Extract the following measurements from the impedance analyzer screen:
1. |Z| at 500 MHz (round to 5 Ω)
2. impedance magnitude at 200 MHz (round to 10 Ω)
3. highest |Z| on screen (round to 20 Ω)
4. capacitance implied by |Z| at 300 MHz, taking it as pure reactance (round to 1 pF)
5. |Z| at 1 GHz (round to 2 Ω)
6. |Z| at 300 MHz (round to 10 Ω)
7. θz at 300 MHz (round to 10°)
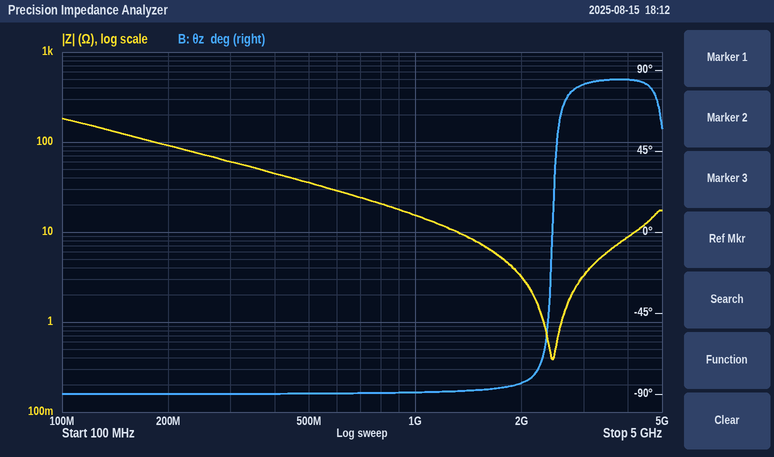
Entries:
35 Ω
90 Ω
180 Ω
9 pF
16 Ω
60 Ω
-90°
